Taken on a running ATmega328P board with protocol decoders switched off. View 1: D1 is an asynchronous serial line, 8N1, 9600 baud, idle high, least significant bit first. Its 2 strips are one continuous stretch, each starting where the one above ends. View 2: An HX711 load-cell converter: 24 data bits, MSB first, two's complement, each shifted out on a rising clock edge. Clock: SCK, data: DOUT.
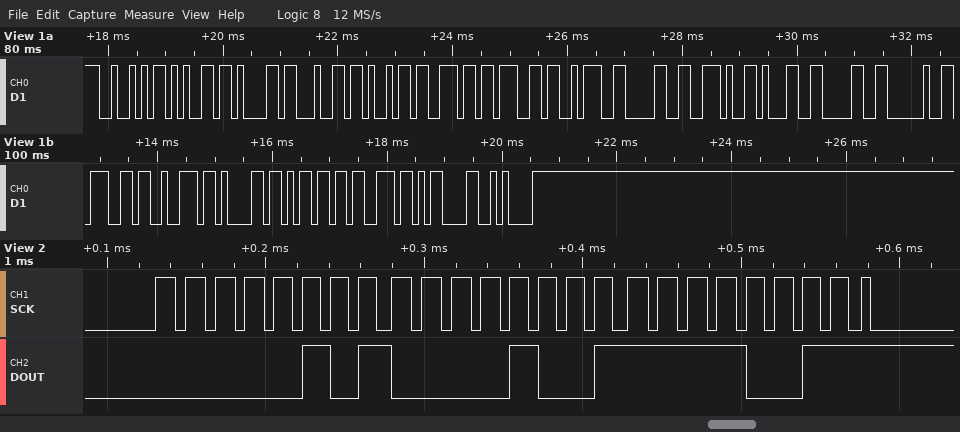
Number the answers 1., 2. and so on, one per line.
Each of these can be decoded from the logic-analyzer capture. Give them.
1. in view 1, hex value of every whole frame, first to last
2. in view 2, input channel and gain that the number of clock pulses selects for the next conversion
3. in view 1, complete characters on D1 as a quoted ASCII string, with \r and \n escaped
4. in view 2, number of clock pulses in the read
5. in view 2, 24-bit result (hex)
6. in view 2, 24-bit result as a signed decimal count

1. 0x52 0x65 0x61 0x64 0x69 0x6E 0x67 0x3A 0x30 0x2E 0x31 0x30 0x20 0x67 0x72 0x61 0x6D 0x73 0x0D 0x0A
2. channel A, gain 128
3. "Reading:0.10 grams\r\n"
4. 25
5. 0x0509F3
6. 330227
